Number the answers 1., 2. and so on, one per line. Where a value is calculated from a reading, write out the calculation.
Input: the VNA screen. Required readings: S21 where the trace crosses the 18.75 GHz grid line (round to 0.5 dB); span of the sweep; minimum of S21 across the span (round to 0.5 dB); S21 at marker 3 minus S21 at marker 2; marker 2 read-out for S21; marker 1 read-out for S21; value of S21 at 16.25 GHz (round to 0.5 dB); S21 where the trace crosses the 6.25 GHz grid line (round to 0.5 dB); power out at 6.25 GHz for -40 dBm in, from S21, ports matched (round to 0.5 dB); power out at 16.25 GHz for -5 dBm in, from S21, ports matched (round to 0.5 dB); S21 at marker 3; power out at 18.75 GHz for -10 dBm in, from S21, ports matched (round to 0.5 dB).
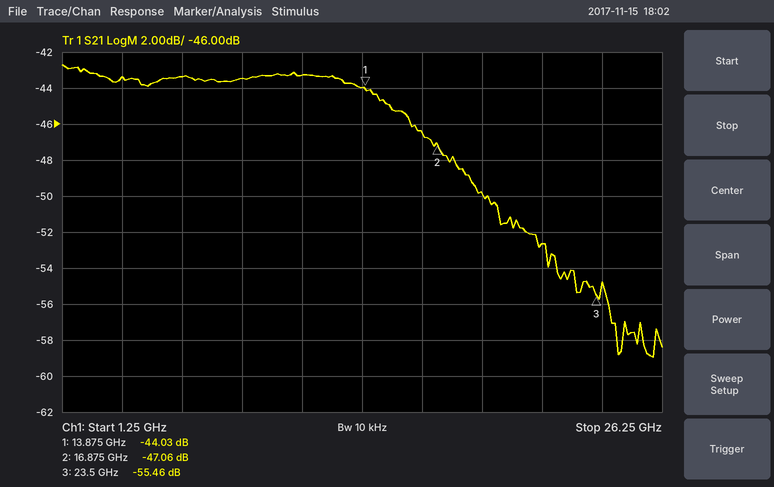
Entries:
1. -50.0 dB
2. 25 GHz
3. -59.0 dB
4. -55.46 − (-47.06) = -8.40 dB
5. -47.06 dB
6. -44.03 dB
7. -46.5 dB
8. -43.5 dB
9. -40 dBm + (-43.5 dB) = -83.5 dBm
10. -5 dBm + (-46.5 dB) = -51.5 dBm
11. -55.46 dB
12. -10 dBm + (-50.0 dB) = -60.0 dBm
